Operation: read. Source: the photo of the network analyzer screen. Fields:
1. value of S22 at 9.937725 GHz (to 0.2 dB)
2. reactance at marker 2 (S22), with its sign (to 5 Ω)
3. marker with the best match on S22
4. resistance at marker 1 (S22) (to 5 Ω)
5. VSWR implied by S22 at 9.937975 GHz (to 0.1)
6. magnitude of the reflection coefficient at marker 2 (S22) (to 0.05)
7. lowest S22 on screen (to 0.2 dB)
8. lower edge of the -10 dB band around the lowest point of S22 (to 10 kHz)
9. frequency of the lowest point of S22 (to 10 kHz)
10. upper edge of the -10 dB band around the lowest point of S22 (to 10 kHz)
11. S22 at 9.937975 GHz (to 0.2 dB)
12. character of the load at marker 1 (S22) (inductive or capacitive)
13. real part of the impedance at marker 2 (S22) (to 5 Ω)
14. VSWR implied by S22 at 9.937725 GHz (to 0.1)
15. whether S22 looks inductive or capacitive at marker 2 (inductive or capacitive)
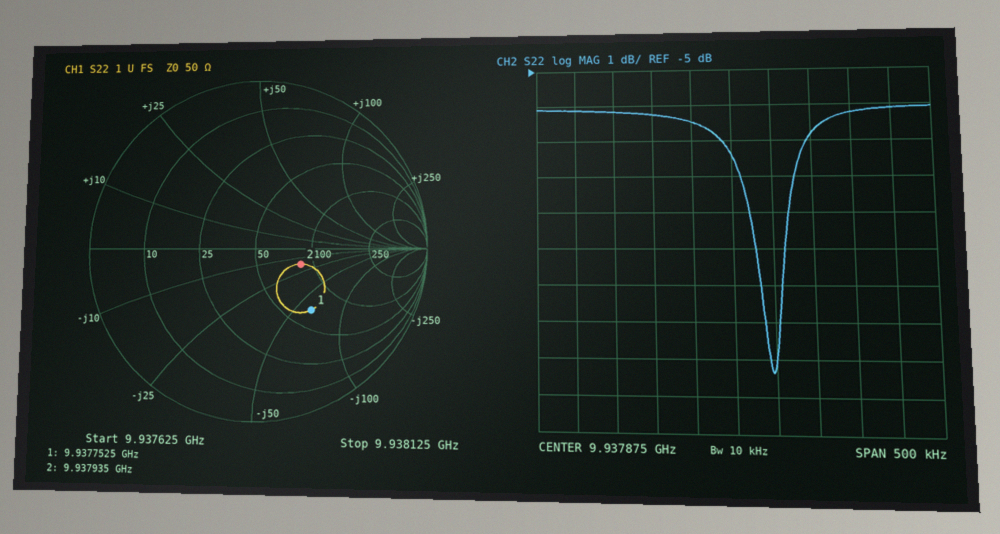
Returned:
-6.2 dB
-15 Ω
marker 2
65 Ω
2.7
0.30
-13.4 dB
9.93790 GHz
9.93792 GHz
9.93794 GHz
-6.8 dB
capacitive
85 Ω
2.9
capacitive
